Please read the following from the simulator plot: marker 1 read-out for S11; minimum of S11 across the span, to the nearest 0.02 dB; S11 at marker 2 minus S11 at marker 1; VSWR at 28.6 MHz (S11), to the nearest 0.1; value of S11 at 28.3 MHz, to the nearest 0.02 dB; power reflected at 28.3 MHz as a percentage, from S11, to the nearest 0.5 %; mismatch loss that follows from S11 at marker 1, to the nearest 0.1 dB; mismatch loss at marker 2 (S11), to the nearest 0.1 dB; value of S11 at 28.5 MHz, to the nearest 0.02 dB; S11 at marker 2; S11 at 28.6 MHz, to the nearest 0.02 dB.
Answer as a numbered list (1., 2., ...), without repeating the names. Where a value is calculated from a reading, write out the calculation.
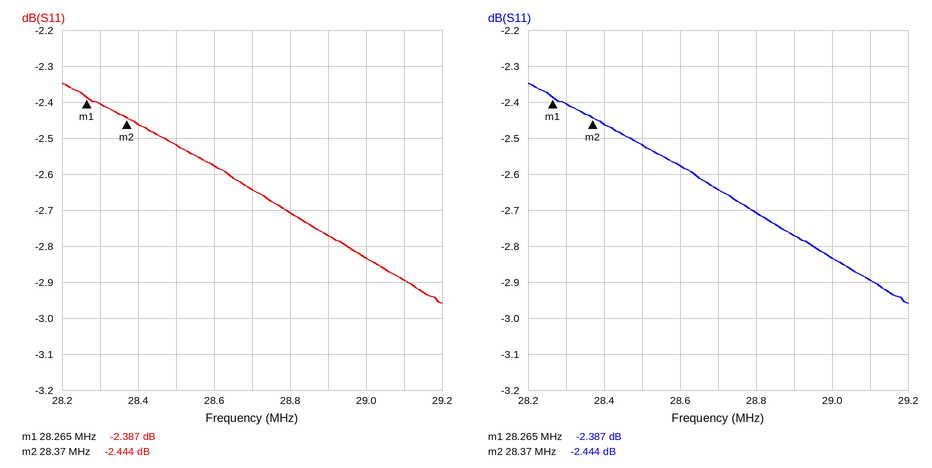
1. -2.387 dB
2. -2.96 dB
3. -2.444 − (-2.387) = -0.057 dB
4. |Γ| = 10^(-2.58/20) = 0.7430; VSWR = (1 + 0.7430)/(1 − 0.7430) ≈ 6.8
5. -2.40 dB
6. 10^(-2.4/10) ≈ 57.5 %
7. −10 log10(1 − 10^(-2.387/10)) ≈ 3.7 dB
8. −10 log10(1 − 10^(-2.444/10)) ≈ 3.7 dB
9. -2.52 dB
10. -2.444 dB
11. -2.58 dB
